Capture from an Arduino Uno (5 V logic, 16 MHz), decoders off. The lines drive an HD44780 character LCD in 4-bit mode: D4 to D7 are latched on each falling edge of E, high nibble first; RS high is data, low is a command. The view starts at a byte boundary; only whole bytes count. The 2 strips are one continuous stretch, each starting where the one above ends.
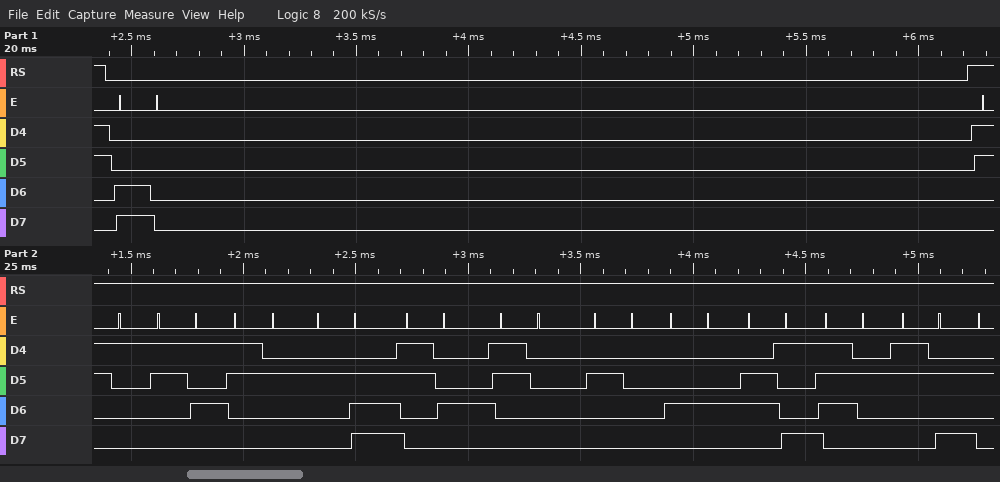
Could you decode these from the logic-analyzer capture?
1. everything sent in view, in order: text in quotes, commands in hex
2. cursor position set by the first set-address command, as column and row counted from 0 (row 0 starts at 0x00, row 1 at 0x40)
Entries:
0xC0 "152.40 Dir:"
column 0, row 1
